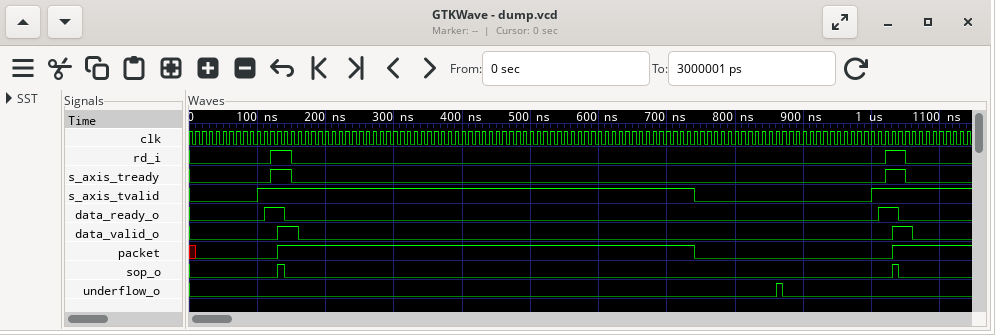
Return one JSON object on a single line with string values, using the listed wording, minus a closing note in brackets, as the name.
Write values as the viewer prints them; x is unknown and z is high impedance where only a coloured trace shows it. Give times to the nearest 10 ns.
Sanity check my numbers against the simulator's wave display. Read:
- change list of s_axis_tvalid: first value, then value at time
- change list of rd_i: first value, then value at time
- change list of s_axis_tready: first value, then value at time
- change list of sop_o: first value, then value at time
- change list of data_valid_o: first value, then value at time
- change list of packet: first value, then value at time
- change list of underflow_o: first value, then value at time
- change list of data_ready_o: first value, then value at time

{"change list of s_axis_tvalid: first value, then value at time": "0, 1 at 100 ns, 0 at 740 ns, 1 at 1000 ns", "change list of rd_i: first value, then value at time": "0, 1 at 120 ns, 0 at 150 ns, 1 at 1020 ns, 0 at 1050 ns", "change list of s_axis_tready: first value, then value at time": "0, 1 at 120 ns, 0 at 150 ns, 1 at 1020 ns, 0 at 1050 ns", "change list of sop_o: first value, then value at time": "0, 1 at 130 ns, 0 at 140 ns, 1 at 1030 ns, 0 at 1040 ns", "change list of data_valid_o: first value, then value at time": "0, 1 at 130 ns, 0 at 160 ns, 1 at 1030 ns, 0 at 1060 ns", "change list of packet: first value, then value at time": "x, 0 at 10 ns, 1 at 130 ns, 0 at 740 ns, 1 at 1030 ns", "change list of underflow_o: first value, then value at time": "0, 1 at 860 ns, 0 at 870 ns", "change list of data_ready_o: first value, then value at time": "0, 1 at 110 ns, 0 at 140 ns, 1 at 1010 ns, 0 at 1040 ns"}
